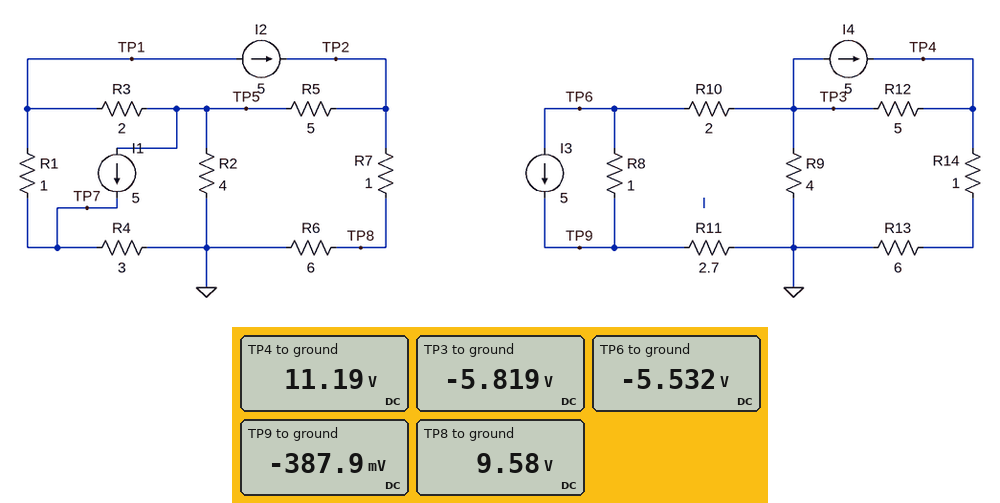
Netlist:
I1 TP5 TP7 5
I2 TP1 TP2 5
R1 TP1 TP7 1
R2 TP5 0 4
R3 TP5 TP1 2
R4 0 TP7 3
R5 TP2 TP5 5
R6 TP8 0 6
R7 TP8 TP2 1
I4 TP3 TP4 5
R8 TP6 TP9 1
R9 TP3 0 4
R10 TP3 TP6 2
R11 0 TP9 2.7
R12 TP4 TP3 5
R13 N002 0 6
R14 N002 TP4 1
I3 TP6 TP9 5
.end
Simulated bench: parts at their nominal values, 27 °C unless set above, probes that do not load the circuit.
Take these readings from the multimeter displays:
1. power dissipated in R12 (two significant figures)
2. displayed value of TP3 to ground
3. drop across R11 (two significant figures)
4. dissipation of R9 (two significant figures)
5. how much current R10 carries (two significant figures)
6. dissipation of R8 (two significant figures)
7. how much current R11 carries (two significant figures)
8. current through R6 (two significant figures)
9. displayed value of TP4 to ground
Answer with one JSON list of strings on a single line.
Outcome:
["58 W", "-5.819 V", "390 mV", "8.5 W", "140 mA", "26 W", "140 mA", "1.6 A", "11.19 V"]
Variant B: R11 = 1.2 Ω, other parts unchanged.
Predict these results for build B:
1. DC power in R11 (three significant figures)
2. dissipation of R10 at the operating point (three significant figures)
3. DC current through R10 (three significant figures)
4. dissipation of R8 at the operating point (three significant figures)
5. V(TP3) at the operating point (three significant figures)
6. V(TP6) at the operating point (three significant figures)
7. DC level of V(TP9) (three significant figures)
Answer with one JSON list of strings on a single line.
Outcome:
["36.2 mW", "60.3 mW", "174 mA", "26.8 W", "-5.73 V", "-5.38 V", "-208 mV"]
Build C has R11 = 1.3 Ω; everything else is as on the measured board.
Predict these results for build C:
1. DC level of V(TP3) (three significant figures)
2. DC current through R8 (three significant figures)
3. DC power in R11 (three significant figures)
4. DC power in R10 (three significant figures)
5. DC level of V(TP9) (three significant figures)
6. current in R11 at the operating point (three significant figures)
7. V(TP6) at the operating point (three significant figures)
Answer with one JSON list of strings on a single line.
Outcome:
["-5.74 V", "5.17 A", "38.1 mW", "58.6 mW", "-223 mV", "171 mA", "-5.39 V"]
